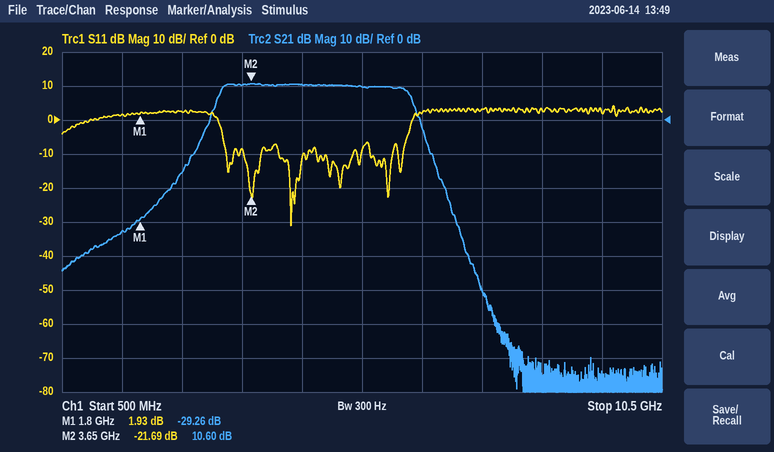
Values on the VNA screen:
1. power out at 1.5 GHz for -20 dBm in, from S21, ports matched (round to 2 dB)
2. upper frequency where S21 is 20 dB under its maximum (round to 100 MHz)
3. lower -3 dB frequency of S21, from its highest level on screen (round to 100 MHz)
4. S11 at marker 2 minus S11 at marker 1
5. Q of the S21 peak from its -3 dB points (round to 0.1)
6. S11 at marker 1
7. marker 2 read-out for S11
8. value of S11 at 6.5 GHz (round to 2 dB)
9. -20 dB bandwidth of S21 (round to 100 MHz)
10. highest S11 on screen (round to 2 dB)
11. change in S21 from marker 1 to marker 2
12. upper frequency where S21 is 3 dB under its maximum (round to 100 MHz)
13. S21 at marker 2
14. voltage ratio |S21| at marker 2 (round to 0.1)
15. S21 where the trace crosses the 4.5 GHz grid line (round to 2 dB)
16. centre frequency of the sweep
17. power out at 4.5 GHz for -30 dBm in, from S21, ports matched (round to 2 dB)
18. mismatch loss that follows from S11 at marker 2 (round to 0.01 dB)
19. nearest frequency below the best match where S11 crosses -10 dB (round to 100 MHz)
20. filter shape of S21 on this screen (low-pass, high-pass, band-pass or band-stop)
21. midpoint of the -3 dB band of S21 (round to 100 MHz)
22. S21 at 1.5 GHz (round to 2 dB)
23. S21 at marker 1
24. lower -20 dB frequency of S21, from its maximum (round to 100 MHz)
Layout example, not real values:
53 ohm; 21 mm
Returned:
-52 dBm; 6.6 GHz; 3.1 GHz; -23.62 dB; 1.5; 1.93 dB; -21.69 dB; 2 dB; 3.9 GHz; 4 dB; 39.86 dB; 6.3 GHz; 10.60 dB; 3.4; 10 dB; 5.5 GHz; -20 dBm; 0.03 dB; 4.1 GHz; band-pass; 4.7 GHz; -32 dB; -29.26 dB; 2.7 GHz
